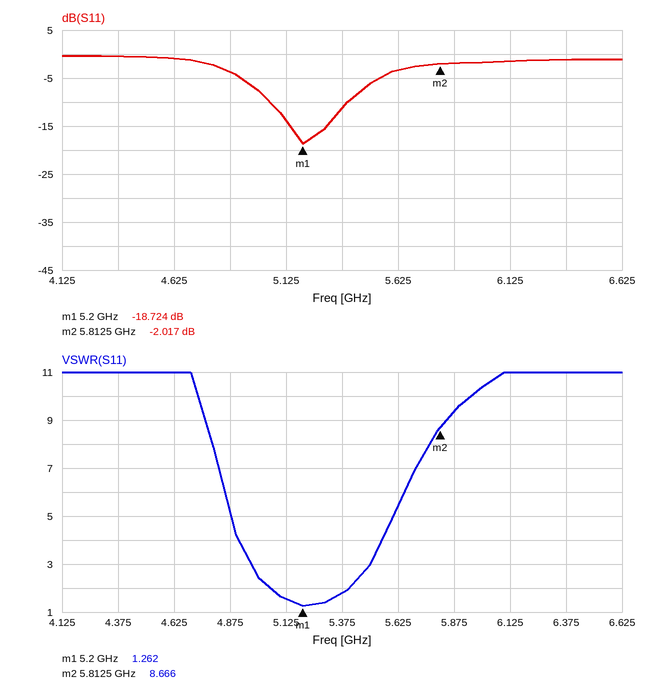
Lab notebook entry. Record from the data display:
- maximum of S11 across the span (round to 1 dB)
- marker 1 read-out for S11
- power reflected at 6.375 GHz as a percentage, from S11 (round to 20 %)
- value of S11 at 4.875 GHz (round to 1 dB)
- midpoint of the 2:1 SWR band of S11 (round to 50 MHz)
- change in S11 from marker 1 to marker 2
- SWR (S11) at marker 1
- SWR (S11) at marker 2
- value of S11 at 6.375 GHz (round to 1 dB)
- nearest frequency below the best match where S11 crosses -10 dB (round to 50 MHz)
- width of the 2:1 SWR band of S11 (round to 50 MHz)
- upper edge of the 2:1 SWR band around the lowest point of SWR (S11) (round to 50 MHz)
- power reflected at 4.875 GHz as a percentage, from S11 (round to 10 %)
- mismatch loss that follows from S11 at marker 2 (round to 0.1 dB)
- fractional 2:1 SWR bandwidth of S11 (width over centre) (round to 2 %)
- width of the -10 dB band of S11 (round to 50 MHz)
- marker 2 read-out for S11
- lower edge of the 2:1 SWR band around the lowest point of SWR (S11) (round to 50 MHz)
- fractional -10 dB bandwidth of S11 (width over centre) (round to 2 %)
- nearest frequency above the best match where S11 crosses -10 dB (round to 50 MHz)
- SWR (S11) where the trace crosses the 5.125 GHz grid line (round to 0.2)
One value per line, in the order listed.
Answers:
0 dB
-18.724 dB
80 %
-4 dB
5.25 GHz
16.707 dB
1.262
8.666
-1 dB
5.05 GHz
350 MHz
5.40 GHz
40 %
4.3 dB
6 %
350 MHz
-2.017 dB
5.05 GHz
6 %
5.40 GHz
1.6
